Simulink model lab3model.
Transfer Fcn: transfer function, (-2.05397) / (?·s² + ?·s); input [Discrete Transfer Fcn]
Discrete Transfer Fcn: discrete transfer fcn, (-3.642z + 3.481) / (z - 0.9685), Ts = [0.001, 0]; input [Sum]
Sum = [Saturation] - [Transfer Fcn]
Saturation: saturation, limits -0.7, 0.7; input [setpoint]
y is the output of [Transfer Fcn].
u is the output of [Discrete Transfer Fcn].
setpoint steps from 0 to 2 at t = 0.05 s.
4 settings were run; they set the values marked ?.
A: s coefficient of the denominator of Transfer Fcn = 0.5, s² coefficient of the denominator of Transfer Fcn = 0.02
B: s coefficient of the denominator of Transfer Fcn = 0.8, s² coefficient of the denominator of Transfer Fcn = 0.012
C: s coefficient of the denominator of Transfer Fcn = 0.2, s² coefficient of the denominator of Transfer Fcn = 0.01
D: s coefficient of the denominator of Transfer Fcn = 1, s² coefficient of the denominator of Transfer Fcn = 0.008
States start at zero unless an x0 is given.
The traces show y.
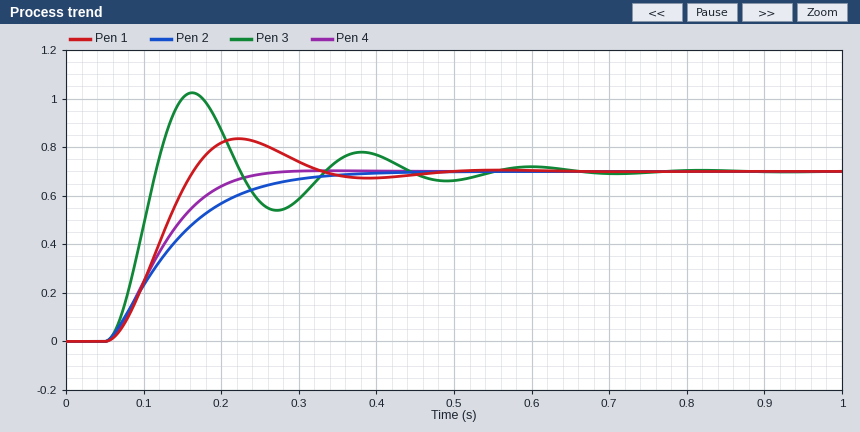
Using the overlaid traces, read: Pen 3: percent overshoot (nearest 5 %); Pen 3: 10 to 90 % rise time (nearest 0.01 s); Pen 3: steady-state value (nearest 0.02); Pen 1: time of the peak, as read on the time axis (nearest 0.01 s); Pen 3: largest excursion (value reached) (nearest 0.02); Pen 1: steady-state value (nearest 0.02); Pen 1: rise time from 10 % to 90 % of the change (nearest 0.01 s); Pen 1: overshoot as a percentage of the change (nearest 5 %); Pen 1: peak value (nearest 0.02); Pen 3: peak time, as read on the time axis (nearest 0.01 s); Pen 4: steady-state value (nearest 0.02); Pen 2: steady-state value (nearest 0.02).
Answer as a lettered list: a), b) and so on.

a) 45 %
b) 0.04 s
c) 0.70
d) 0.22 s
e) 1.02
f) 0.70
g) 0.08 s
h) 20 %
i) 0.84
j) 0.16 s
k) 0.70
l) 0.70
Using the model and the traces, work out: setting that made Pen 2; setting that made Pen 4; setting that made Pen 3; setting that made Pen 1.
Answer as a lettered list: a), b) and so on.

a) D
b) B
c) C
d) A
